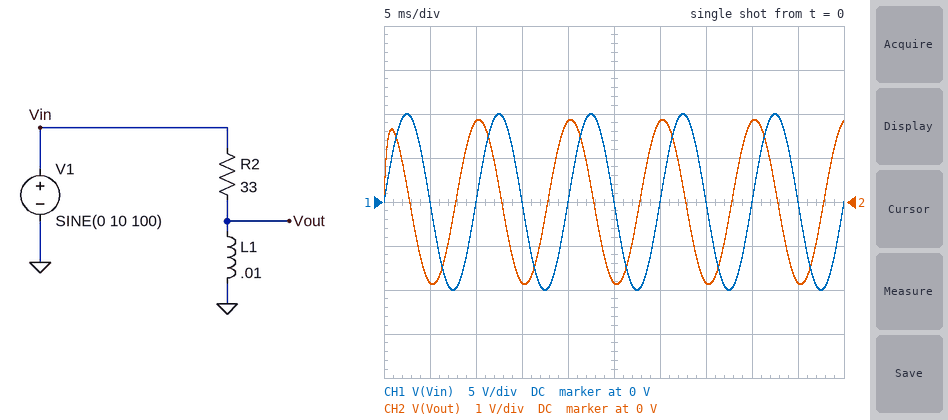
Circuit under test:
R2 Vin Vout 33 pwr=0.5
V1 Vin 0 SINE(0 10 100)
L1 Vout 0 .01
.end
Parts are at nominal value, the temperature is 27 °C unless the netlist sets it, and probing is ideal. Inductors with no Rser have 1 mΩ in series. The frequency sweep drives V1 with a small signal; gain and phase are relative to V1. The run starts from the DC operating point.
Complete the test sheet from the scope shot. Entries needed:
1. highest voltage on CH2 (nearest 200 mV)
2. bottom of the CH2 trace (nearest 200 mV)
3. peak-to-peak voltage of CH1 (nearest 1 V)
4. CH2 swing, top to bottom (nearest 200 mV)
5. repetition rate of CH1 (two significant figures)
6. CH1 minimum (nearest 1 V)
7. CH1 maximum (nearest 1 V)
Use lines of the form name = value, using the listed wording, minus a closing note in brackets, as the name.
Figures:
highest voltage on CH2 = 1.8 V
bottom of the CH2 trace = -1.8 V
peak-to-peak voltage of CH1 = 20 V
CH2 swing, top to bottom = 3.8 V
repetition rate of CH1 = 100 Hz
CH1 minimum = -10 V
CH1 maximum = 10 V
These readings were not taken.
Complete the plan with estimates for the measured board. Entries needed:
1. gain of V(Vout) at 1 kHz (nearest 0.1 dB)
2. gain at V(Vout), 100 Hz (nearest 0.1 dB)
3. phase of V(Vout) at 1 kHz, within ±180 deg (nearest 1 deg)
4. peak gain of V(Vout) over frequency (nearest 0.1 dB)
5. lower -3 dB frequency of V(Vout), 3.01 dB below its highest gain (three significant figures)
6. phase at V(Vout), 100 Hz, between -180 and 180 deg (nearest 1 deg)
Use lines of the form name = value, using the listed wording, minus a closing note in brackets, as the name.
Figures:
gain of V(Vout) at 1 kHz = -1.1 dB
gain at V(Vout), 100 Hz = -14.6 dB
phase of V(Vout) at 1 kHz, within ±180 deg = 28 deg
peak gain of V(Vout) over frequency = 0 dB
lower -3 dB frequency of V(Vout), 3.01 dB below its highest gain = 525 Hz
phase at V(Vout), 100 Hz, between -180 and 180 deg = 79 deg
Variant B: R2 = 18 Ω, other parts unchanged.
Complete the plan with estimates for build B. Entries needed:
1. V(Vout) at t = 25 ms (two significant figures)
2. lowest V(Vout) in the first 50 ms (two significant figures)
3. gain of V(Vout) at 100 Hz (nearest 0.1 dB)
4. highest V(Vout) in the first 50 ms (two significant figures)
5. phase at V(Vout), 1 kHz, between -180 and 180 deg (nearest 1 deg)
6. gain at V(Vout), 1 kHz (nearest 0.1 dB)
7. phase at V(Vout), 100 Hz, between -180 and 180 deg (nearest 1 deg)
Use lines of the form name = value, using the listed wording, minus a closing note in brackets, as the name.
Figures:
V(Vout) at t = 25 ms = -3.1 V
lowest V(Vout) in the first 50 ms = -3.3 V
gain of V(Vout) at 100 Hz = -9.6 dB
highest V(Vout) in the first 50 ms = 3.3 V
phase at V(Vout), 1 kHz, between -180 and 180 deg = 16 deg
gain at V(Vout), 1 kHz = -0.3 dB
phase at V(Vout), 100 Hz, between -180 and 180 deg = 71 deg
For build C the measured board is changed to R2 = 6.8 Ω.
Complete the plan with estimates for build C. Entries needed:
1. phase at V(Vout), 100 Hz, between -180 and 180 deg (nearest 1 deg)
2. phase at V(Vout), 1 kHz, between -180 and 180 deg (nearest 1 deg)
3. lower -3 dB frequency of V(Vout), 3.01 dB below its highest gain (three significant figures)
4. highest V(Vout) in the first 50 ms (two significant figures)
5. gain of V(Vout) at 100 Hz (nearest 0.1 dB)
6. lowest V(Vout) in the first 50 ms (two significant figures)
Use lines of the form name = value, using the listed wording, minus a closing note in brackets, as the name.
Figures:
phase at V(Vout), 100 Hz, between -180 and 180 deg = 47 deg
phase at V(Vout), 1 kHz, between -180 and 180 deg = 6 deg
lower -3 dB frequency of V(Vout), 3.01 dB below its highest gain = 108 Hz
highest V(Vout) in the first 50 ms = 6.8 V
gain of V(Vout) at 100 Hz = -3.4 dB
lowest V(Vout) in the first 50 ms = -6.9 V
